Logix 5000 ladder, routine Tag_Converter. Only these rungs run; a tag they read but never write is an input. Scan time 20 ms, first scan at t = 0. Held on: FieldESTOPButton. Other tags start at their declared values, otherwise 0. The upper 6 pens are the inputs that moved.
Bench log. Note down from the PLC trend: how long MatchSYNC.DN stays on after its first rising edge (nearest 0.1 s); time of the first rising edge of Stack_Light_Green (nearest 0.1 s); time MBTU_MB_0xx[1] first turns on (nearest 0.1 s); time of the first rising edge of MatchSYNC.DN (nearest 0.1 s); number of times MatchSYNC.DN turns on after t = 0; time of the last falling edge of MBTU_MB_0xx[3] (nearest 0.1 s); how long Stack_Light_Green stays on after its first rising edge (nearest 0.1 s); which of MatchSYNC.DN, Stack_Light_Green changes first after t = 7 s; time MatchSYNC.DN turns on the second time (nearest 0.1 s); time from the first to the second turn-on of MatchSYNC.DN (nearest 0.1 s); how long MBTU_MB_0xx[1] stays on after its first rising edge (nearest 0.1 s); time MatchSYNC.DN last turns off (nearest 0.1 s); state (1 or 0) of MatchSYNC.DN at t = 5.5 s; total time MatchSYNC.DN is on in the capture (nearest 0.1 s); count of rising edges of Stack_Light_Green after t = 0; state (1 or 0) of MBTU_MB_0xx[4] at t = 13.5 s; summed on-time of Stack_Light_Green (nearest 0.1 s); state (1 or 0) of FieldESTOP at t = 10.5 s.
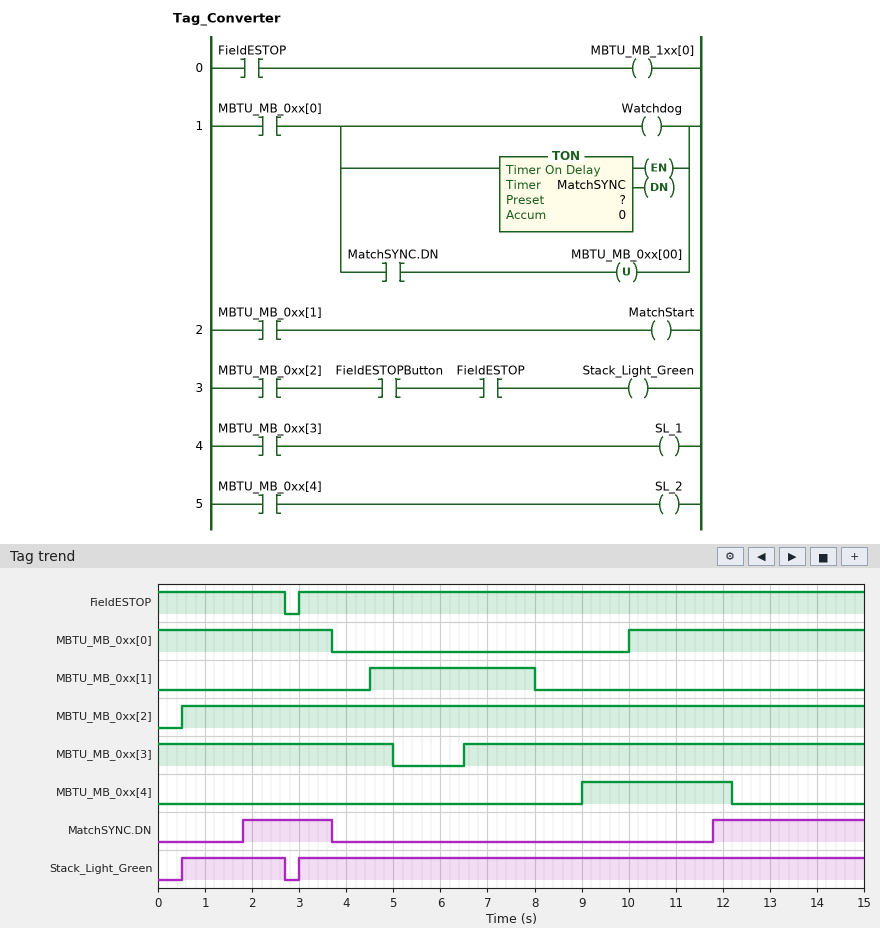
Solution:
1.9 s
0.5 s
4.5 s
1.8 s
2
5.0 s
2.2 s
MatchSYNC.DN
11.8 s
10.0 s
3.5 s
3.7 s
0
5.1 s
2
0
14.2 s
1
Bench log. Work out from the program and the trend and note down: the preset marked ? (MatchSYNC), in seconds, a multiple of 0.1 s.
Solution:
1.8 s
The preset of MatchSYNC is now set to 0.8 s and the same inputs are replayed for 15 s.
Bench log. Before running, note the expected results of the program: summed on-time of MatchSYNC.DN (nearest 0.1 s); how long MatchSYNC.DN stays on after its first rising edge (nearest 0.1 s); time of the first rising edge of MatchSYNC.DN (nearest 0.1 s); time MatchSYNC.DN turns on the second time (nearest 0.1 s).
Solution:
7.1 s
2.9 s
0.8 s
10.8 s
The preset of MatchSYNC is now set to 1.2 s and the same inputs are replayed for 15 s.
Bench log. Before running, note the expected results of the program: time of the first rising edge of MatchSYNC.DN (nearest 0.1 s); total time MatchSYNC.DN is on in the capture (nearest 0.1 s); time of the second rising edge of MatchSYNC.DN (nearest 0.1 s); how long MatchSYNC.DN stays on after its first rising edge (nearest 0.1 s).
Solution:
1.2 s
6.3 s
11.2 s
2.5 s
